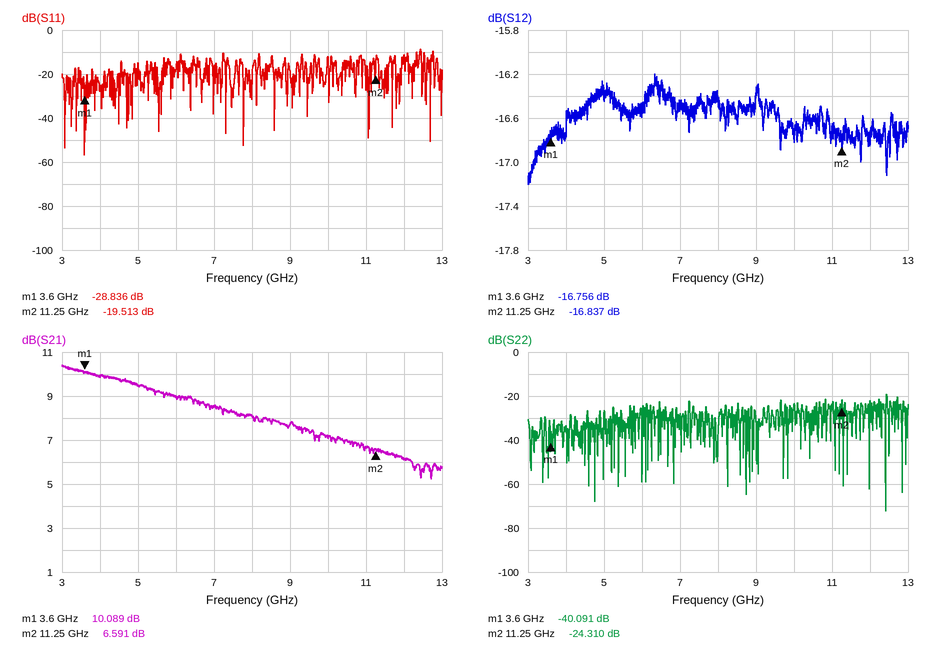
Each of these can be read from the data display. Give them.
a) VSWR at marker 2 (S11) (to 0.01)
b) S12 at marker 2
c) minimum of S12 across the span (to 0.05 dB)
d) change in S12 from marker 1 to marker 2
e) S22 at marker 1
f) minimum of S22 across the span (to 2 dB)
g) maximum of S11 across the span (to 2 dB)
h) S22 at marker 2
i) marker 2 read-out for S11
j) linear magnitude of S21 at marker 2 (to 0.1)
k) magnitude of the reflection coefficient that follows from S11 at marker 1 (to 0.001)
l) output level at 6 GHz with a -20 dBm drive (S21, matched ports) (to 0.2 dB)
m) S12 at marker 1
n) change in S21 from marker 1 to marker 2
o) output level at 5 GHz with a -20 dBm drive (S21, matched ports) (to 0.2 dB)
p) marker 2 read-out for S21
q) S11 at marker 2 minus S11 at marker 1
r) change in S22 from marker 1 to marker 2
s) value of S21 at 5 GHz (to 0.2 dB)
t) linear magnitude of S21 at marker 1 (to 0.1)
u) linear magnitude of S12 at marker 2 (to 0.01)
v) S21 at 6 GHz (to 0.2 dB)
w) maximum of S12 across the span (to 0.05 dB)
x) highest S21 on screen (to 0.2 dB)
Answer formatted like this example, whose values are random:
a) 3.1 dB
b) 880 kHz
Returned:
a) 1.24
b) -16.837 dB
c) -17.20 dB
d) -0.081 dB
e) -40.091 dB
f) -72 dB
g) -8 dB
h) -24.310 dB
i) -19.513 dB
j) 2.1
k) 0.036
l) -11.0 dBm
m) -16.756 dB
n) -3.498 dB
o) -10.6 dBm
p) 6.591 dB
q) 9.323 dB
r) 15.781 dB
s) 9.4 dB
t) 3.2
u) 0.14
v) 9.0 dB
w) -16.20 dB
x) 10.4 dB
